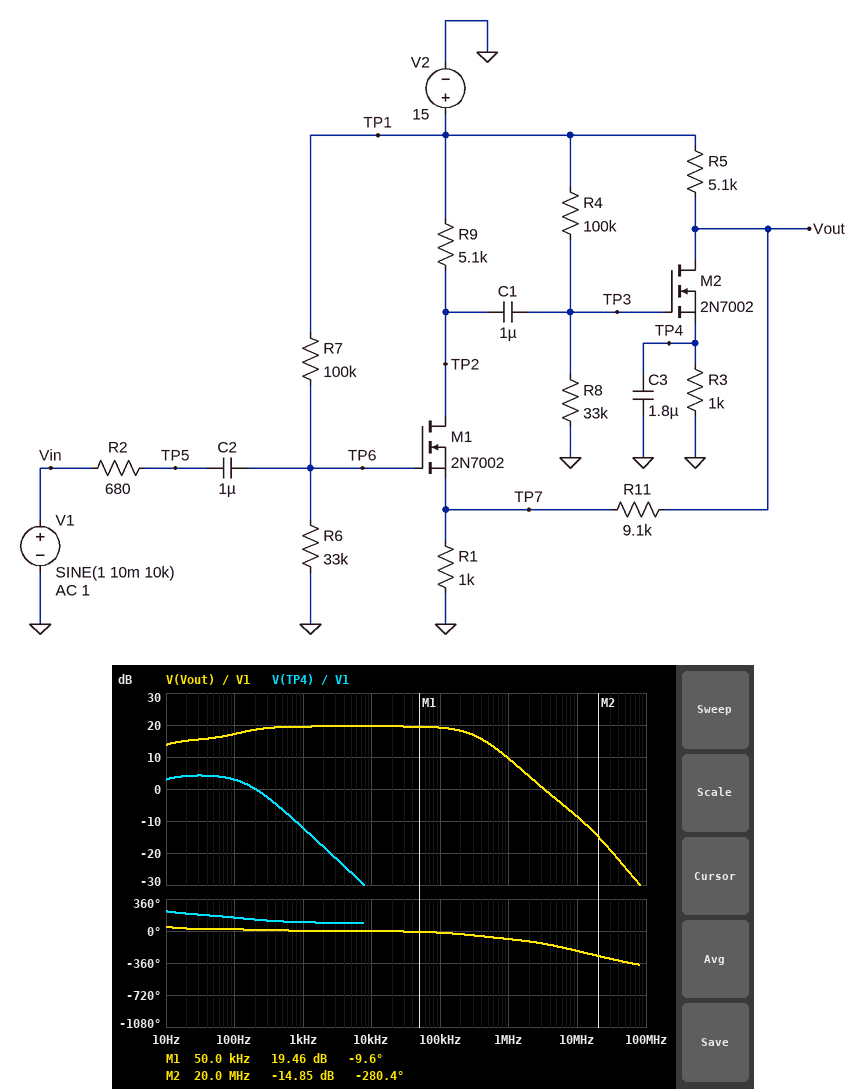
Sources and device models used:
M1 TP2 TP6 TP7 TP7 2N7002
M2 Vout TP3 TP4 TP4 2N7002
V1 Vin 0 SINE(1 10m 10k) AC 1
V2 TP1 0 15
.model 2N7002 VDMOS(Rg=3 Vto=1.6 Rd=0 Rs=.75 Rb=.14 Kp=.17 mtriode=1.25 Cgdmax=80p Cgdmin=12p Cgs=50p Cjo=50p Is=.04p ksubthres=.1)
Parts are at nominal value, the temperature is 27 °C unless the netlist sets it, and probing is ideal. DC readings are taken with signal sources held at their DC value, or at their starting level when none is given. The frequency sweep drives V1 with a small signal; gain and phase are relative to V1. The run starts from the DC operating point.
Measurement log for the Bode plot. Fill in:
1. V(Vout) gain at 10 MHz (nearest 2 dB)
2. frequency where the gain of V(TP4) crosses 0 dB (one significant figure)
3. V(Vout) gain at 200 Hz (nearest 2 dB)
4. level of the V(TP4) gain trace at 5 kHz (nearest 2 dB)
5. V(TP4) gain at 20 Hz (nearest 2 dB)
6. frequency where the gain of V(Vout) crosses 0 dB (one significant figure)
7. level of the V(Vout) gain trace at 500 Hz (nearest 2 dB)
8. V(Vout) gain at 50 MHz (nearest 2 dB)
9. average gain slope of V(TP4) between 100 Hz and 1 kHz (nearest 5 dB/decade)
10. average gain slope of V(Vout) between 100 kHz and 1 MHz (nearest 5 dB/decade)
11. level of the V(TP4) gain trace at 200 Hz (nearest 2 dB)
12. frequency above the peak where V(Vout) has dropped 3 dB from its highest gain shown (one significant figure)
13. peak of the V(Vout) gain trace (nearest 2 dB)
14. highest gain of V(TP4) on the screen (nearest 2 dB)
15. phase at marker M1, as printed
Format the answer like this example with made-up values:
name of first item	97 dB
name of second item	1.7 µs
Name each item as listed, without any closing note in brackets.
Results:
V(Vout) gain at 10 MHz	-8 dB
frequency where the gain of V(TP4) crosses 0 dB	200 Hz
V(Vout) gain at 200 Hz	18 dB
level of the V(TP4) gain trace at 5 kHz	-26 dB
V(TP4) gain at 20 Hz	4 dB
frequency where the gain of V(Vout) crosses 0 dB	3 MHz
level of the V(Vout) gain trace at 500 Hz	20 dB
V(Vout) gain at 50 MHz	-24 dB
average gain slope of V(TP4) between 100 Hz and 1 kHz	-15 dB/decade
average gain slope of V(Vout) between 100 kHz and 1 MHz	-10 dB/decade
level of the V(TP4) gain trace at 200 Hz	0 dB
frequency above the peak where V(Vout) has dropped 3 dB from its highest gain shown	300 kHz
peak of the V(Vout) gain trace	20 dB
highest gain of V(TP4) on the screen	4 dB
phase at marker M1, as printed	-9.6 deg
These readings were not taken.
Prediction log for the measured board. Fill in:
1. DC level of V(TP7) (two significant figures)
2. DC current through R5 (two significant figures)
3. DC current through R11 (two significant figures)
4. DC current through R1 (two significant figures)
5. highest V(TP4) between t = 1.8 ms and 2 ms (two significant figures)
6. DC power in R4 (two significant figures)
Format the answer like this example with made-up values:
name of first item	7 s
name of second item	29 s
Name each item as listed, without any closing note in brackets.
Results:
DC level of V(TP7)	2.0 V
DC current through R5	2.2 mA
DC current through R11	200 µA
DC current through R1	2.0 mA
highest V(TP4) between t = 1.8 ms and 2 ms	2.0 V
DC power in R4	1.3 mW
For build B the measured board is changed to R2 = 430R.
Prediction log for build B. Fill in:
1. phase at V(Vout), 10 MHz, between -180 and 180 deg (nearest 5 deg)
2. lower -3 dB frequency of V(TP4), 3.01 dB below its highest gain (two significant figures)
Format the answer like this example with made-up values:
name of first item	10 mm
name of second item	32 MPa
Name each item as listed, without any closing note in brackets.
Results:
phase at V(Vout), 10 MHz, between -180 and 180 deg	145 deg
lower -3 dB frequency of V(TP4), 3.01 dB below its highest gain	6.5 Hz
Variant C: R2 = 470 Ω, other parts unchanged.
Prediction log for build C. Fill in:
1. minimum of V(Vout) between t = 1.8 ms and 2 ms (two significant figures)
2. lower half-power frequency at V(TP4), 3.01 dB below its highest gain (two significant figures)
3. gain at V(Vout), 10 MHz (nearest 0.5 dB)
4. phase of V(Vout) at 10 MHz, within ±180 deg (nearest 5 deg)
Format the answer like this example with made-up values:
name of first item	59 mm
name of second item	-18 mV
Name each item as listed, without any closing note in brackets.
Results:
minimum of V(Vout) between t = 1.8 ms and 2 ms	3.7 V
lower half-power frequency at V(TP4), 3.01 dB below its highest gain	6.5 Hz
gain at V(Vout), 10 MHz	-7.0 dB
phase of V(Vout) at 10 MHz, within ±180 deg	145 deg
